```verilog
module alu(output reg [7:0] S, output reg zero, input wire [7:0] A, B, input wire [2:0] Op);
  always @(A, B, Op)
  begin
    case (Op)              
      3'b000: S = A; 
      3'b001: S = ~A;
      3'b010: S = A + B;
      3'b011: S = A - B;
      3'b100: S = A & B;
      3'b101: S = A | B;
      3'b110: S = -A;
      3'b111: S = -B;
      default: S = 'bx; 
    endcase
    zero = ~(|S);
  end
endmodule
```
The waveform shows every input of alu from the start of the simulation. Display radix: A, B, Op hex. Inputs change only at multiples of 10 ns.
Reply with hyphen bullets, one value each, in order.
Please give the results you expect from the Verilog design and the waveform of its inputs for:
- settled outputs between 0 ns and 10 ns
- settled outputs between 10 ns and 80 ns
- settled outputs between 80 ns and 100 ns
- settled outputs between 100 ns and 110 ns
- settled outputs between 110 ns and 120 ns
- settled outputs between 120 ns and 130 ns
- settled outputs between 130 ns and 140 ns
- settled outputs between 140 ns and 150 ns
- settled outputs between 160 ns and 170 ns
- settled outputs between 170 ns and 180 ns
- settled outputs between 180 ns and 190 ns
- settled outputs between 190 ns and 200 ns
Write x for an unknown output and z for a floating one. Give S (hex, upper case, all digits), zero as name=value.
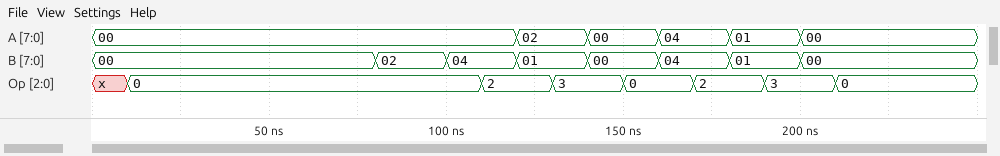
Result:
- S=x, zero=x
- S=00, zero=1
- S=00, zero=1
- S=00, zero=1
- S=04, zero=0
- S=03, zero=0
- S=01, zero=0
- S=00, zero=1
- S=04, zero=0
- S=08, zero=0
- S=02, zero=0
- S=00, zero=1
